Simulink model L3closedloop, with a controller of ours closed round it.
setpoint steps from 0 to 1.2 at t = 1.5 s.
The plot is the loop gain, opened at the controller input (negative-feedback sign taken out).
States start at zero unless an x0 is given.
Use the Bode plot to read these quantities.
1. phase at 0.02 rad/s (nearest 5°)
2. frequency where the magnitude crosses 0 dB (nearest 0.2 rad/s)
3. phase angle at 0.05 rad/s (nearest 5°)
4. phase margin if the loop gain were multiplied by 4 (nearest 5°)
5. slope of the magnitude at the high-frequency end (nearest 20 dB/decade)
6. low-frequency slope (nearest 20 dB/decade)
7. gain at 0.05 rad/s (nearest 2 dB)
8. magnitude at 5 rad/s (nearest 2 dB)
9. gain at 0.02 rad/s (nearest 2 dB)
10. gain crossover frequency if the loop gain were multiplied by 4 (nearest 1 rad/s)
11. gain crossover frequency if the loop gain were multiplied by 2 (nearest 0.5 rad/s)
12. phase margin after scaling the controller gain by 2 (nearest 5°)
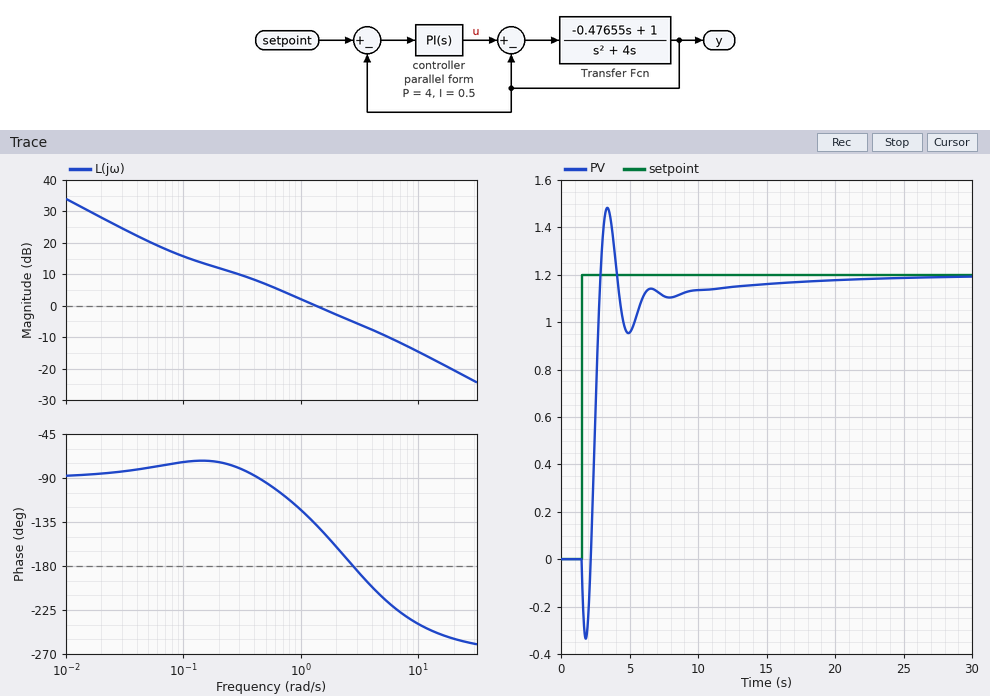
-85°
1.4 rad/s
-80°
-50°
-20 dB/decade
-20 dB/decade
20 dB
-10 dB
28 dB
7 rad/s
3.0 rad/s
-10°
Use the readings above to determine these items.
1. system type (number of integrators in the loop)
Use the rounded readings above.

1
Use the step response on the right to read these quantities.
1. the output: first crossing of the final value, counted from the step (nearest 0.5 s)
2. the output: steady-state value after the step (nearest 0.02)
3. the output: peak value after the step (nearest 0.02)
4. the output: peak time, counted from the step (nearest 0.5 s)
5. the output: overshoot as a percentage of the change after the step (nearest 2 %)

1.5 s
1.20
1.48
2.0 s
24 %
